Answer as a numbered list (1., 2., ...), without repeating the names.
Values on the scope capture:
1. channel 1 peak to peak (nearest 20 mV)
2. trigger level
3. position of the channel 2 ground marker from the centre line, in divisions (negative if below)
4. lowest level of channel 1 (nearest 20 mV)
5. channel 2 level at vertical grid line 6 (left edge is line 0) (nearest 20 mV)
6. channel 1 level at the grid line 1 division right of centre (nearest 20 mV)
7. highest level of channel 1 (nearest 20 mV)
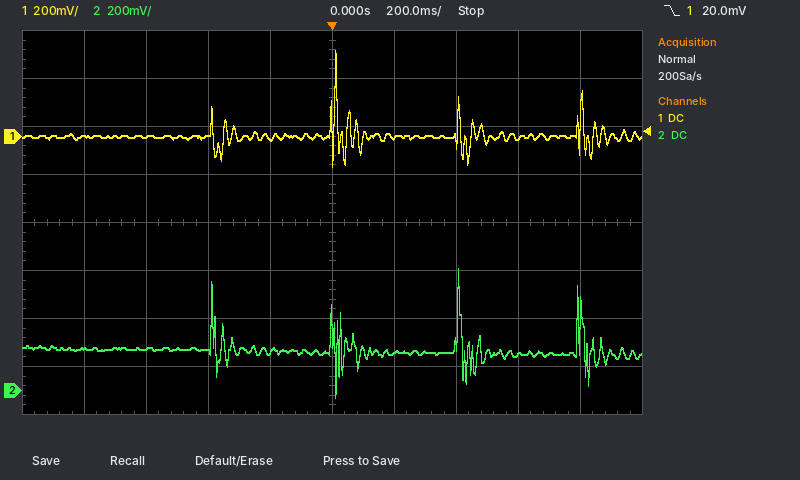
1. 480 mV
2. 20.0 mV
3. -3.5 div
4. -120 mV
5. 160 mV
6. 0 mV
7. 360 mV
